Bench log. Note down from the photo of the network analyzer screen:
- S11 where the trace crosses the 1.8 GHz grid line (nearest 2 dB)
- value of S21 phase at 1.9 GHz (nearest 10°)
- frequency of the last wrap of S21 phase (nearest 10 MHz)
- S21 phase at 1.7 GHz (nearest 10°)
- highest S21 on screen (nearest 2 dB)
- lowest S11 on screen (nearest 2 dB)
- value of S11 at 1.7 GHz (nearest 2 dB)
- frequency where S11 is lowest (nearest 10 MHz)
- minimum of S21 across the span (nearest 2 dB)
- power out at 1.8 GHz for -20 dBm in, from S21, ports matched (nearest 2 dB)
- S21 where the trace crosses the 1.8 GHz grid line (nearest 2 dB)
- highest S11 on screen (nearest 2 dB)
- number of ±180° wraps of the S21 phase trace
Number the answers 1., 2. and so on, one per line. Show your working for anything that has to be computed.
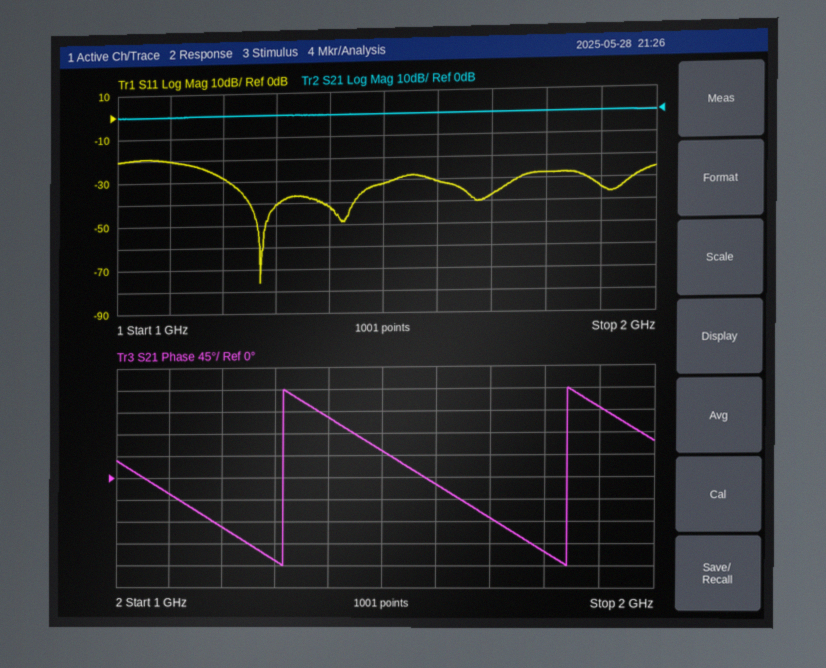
1. -28 dB
2. 140°
3. 1.84 GHz
4. -80°
5. 0 dB
6. -76 dB
7. -38 dB
8. 1.27 GHz
9. 0 dB
10. -20 dBm + (0 dB) = -20 dBm
11. 0 dB
12. -20 dB
13. 2
